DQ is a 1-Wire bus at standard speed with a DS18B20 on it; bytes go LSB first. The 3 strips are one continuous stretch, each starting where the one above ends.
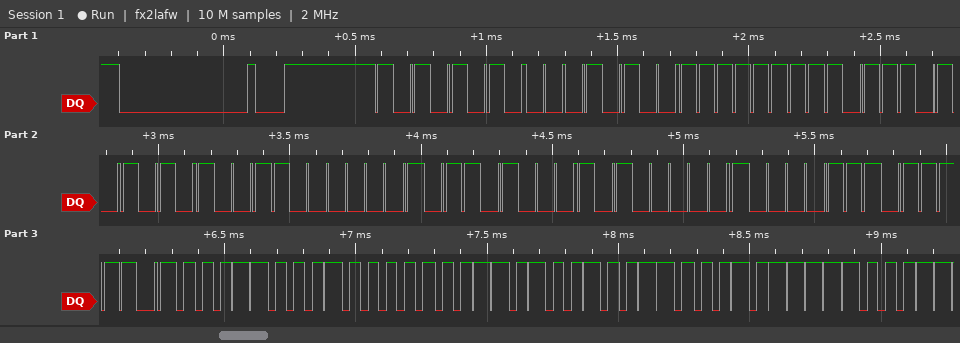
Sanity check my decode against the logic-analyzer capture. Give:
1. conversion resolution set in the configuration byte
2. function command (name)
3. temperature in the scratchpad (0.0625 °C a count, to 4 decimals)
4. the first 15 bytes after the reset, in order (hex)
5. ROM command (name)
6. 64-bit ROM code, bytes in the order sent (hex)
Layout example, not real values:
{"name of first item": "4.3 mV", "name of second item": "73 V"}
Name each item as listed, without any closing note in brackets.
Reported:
{"conversion resolution set in the configuration byte": "9 bits", "function command": "Read Scratchpad", "temperature in the scratchpad": "17.5000 °C", "the first 15 bytes after the reset, in order": "55 28 FF 5D 95 81 16 05 E1 BE 18 01 4B 46 1F", "ROM command": "Match ROM", "64-bit ROM code, bytes in the order sent": "28 FF 5D 95 81 16 05 E1"}
